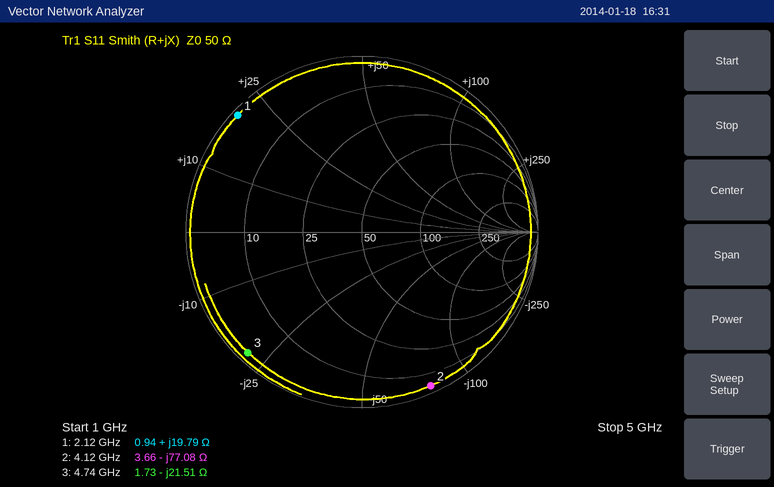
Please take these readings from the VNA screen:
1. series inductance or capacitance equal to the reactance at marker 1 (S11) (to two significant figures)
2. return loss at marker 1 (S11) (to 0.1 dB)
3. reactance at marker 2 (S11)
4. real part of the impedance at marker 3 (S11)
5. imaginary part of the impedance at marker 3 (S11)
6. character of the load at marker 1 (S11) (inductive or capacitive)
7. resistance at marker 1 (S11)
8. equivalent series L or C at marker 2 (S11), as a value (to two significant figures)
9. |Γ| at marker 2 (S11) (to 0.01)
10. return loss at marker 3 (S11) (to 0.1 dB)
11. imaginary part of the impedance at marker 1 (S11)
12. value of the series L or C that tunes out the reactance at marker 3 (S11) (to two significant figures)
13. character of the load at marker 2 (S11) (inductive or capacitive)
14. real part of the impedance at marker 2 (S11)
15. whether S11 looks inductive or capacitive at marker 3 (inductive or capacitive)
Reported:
1.5 nH
0.3 dB
-77.08 Ω
1.73 Ω
-21.51 Ω
inductive
0.94 Ω
500 fF
0.96
0.5 dB
+19.79 Ω
720 pH
capacitive
3.66 Ω
capacitive
